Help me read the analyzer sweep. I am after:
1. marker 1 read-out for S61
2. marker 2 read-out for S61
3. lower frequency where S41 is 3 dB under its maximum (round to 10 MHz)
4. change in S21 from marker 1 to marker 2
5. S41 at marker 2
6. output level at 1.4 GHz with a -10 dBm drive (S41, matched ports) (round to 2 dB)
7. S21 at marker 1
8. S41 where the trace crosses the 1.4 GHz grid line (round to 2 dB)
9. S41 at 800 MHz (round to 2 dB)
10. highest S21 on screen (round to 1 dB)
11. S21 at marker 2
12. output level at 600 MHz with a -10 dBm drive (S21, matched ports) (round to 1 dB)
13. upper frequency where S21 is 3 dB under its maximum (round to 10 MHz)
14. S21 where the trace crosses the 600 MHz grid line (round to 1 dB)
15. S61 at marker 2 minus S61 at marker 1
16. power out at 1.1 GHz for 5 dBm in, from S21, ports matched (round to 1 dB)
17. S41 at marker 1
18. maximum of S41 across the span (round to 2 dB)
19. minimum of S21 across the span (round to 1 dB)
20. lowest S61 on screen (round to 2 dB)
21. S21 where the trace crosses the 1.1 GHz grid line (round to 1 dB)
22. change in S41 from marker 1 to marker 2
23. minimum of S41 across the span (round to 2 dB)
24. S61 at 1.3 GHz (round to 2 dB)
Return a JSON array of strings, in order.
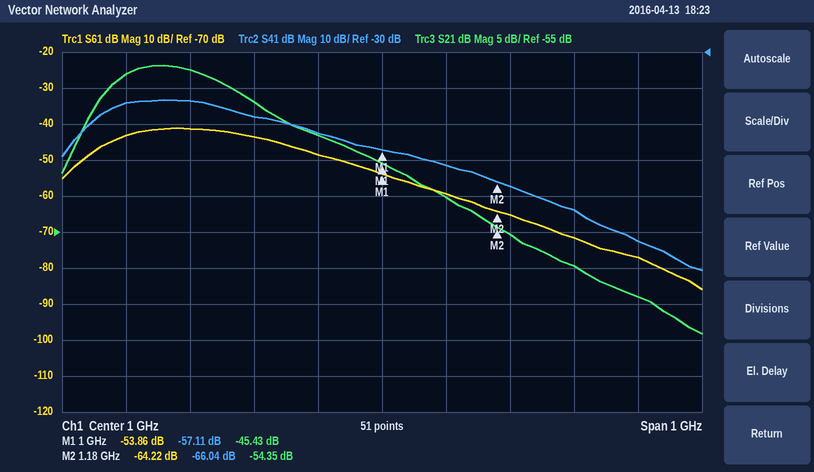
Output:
["-53.86 dB", "-64.22 dB", "570 MHz", "-8.92 dB", "-66.04 dB", "-92 dBm", "-45.43 dB", "-82 dB", "-48 dB", "-32 dB", "-54.35 dB", "-43 dBm", "760 MHz", "-33 dB", "-10.36 dB", "-45 dBm", "-57.11 dB", "-44 dB", "-69 dB", "-86 dB", "-50 dB", "-8.93 dB", "-90 dB", "-72 dB"]
